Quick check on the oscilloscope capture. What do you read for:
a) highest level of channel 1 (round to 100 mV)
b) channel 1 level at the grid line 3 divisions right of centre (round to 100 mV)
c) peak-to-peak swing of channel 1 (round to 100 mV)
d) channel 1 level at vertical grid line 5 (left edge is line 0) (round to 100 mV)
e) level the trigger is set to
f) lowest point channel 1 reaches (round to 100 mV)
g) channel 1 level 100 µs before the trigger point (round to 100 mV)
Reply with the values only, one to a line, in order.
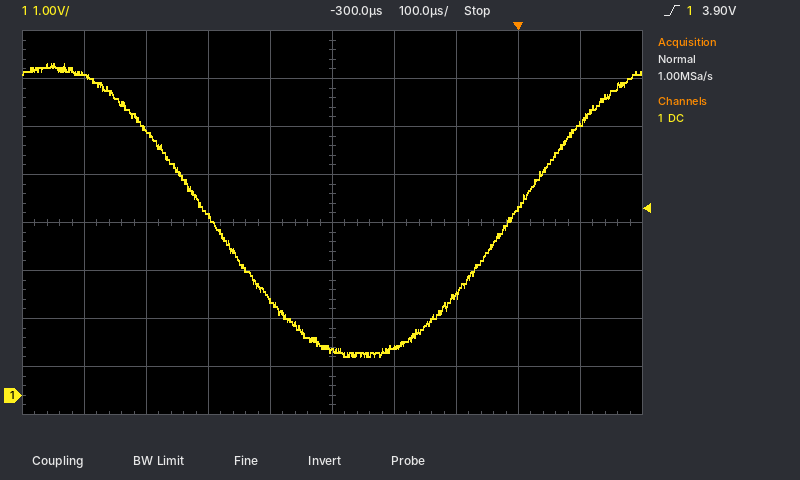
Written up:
6.9 V
3.9 V
6.1 V
900 mV
3.90 V
800 mV
2.1 V
